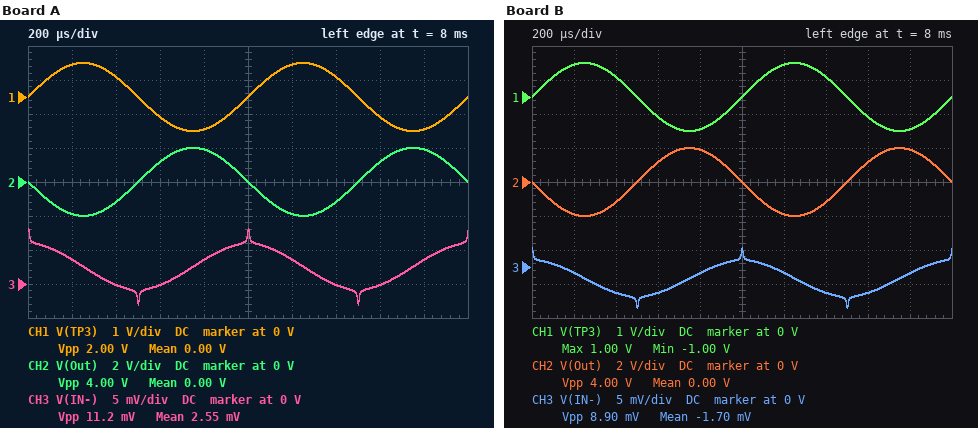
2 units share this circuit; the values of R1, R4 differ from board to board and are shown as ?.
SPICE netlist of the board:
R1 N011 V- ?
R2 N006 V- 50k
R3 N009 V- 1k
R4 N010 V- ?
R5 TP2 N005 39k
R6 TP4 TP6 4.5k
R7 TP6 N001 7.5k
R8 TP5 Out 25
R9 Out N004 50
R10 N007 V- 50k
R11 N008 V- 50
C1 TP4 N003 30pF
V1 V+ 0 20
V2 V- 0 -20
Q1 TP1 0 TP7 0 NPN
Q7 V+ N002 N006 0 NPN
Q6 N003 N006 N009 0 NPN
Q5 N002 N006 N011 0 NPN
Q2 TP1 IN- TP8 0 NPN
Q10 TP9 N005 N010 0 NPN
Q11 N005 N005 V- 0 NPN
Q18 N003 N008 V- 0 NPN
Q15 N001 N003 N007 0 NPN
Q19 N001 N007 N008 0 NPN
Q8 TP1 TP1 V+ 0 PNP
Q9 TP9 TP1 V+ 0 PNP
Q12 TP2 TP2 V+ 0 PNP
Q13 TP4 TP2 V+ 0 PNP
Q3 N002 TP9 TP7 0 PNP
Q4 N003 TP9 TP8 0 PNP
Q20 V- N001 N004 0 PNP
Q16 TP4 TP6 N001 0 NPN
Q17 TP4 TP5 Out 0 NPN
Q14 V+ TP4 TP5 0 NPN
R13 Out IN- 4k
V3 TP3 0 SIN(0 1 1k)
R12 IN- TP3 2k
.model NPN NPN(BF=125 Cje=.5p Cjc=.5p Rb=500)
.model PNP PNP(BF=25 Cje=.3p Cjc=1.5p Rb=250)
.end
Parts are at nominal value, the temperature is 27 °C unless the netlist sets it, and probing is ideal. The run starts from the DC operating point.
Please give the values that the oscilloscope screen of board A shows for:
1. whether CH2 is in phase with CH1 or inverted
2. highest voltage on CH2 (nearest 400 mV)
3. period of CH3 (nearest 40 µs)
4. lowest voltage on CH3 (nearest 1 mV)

inverted
2.0 V
1.00 ms
-3 mV
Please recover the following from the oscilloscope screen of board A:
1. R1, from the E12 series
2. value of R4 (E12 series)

1.2 kΩ
10 kΩ
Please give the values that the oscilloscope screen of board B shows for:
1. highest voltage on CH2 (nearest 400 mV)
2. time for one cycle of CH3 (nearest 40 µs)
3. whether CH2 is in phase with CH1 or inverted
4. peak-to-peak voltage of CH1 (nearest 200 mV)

2.0 V
1.00 ms
inverted
2.0 V
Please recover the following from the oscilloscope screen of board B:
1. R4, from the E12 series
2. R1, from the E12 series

6.8 kΩ
820 Ω
